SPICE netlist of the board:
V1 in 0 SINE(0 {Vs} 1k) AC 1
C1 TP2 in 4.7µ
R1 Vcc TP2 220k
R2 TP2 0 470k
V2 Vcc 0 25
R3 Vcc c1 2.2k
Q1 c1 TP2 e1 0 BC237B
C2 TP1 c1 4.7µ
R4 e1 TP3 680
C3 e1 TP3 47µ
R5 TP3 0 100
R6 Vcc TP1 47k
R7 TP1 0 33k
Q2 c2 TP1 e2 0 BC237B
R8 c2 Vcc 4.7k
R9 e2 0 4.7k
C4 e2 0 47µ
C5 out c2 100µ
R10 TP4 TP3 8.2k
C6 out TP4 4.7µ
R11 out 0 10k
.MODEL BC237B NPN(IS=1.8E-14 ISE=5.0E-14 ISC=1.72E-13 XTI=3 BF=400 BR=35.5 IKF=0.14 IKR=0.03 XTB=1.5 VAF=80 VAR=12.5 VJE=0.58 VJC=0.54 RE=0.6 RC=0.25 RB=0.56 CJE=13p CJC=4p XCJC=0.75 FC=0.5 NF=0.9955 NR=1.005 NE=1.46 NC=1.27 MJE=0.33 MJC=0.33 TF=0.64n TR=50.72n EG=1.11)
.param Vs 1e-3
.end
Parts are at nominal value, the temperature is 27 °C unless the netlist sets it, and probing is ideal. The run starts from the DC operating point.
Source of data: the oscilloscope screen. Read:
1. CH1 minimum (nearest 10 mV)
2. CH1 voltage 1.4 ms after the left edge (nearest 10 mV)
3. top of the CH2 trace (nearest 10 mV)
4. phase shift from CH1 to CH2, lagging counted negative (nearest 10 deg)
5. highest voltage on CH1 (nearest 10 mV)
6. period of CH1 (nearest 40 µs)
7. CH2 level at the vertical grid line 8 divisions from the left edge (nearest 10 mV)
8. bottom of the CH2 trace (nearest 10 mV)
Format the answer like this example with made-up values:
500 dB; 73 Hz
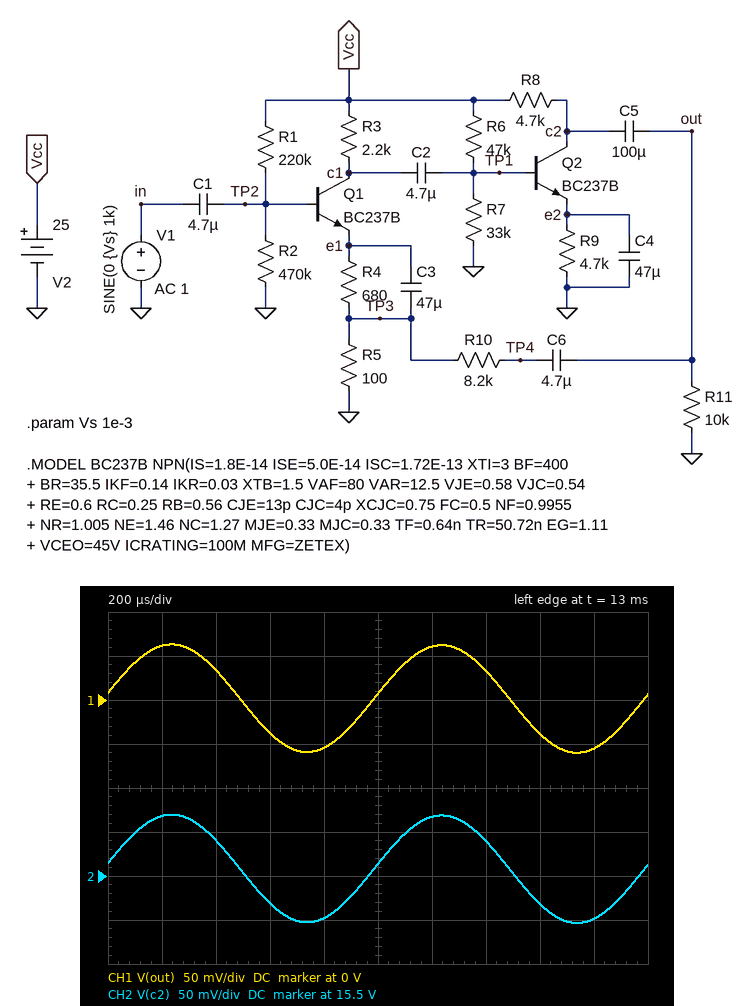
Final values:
-60 mV; 30 mV; 15.57 V; 0 deg; 60 mV; 1.00 ms; 15.47 V; 15.45 V
